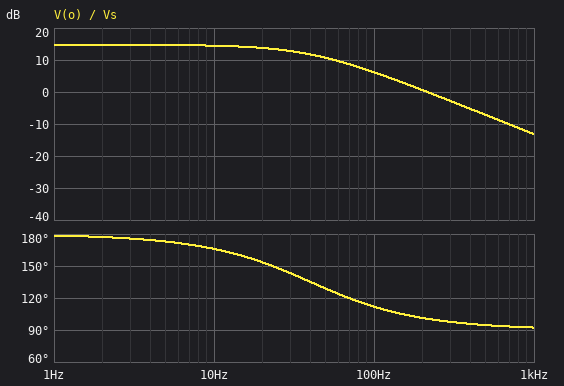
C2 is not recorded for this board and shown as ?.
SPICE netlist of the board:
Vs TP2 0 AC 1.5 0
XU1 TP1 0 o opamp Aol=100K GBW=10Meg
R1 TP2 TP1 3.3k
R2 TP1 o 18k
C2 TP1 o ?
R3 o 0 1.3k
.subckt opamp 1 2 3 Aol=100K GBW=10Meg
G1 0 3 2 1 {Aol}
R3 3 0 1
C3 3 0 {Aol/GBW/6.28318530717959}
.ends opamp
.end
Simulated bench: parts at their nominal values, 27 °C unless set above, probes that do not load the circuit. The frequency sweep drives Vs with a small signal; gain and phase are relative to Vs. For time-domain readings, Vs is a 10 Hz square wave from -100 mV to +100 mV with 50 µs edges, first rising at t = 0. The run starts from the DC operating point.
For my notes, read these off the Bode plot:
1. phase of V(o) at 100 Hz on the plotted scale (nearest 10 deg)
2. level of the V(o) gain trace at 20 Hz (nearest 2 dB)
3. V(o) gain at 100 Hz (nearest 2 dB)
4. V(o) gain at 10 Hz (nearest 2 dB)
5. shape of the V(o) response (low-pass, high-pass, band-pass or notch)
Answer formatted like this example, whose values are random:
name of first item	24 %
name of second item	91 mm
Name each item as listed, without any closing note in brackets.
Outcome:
phase of V(o) at 100 Hz on the plotted scale	110 deg
level of the V(o) gain trace at 20 Hz	14 dB
V(o) gain at 100 Hz	6 dB
V(o) gain at 10 Hz	14 dB
shape of the V(o) response	low-pass
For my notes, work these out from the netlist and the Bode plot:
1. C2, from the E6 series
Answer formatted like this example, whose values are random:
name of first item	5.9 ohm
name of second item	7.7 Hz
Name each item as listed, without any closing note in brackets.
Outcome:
C2, from the E6 series	220 nF
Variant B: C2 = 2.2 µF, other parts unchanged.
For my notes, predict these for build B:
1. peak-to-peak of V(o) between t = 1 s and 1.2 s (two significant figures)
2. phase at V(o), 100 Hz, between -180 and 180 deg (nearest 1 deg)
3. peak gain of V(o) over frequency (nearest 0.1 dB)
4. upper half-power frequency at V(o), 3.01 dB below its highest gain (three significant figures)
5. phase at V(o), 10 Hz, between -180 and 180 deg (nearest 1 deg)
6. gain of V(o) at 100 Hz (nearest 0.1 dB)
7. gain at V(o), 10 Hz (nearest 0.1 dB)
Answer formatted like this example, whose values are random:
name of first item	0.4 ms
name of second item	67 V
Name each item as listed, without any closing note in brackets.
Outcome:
peak-to-peak of V(o) between t = 1 s and 1.2 s	610 mV
phase at V(o), 100 Hz, between -180 and 180 deg	92 deg
peak gain of V(o) over frequency	14.7 dB
upper half-power frequency at V(o), 3.01 dB below its highest gain	4.02 Hz
phase at V(o), 10 Hz, between -180 and 180 deg	112 deg
gain of V(o) at 100 Hz	-13.2 dB
gain at V(o), 10 Hz	6.2 dB
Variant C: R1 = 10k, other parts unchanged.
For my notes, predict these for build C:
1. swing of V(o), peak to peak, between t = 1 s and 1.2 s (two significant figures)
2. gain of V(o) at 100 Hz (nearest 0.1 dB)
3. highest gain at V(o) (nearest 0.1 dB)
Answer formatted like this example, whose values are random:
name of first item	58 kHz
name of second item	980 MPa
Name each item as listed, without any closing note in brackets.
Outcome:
swing of V(o), peak to peak, between t = 1 s and 1.2 s	360 mV
gain of V(o) at 100 Hz	-3.5 dB
highest gain at V(o)	5.1 dB
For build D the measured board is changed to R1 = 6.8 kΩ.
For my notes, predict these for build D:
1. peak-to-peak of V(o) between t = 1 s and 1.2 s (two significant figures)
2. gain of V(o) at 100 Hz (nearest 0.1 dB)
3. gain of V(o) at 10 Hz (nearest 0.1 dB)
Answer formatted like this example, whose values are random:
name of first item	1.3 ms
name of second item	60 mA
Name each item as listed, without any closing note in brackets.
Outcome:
peak-to-peak of V(o) between t = 1 s and 1.2 s	530 mV
gain of V(o) at 100 Hz	-0.1 dB
gain of V(o) at 10 Hz	8.2 dB
